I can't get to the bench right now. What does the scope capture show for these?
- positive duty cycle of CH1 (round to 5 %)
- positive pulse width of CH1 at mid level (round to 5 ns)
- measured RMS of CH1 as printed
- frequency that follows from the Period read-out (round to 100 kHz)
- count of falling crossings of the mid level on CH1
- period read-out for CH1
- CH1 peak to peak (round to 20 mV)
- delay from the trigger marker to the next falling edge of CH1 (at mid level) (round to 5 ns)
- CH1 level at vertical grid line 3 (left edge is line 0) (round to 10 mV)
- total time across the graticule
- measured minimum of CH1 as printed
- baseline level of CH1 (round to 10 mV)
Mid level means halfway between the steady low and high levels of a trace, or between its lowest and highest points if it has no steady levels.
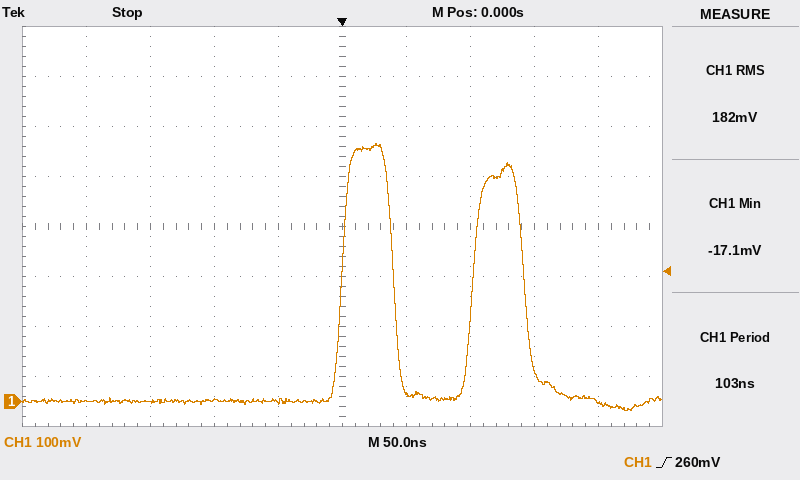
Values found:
40 %
40 ns
182 mV
9.7 MHz
2
103 ns
540 mV
40 ns
0 mV
500 ns
-17.1 mV
0 mV
